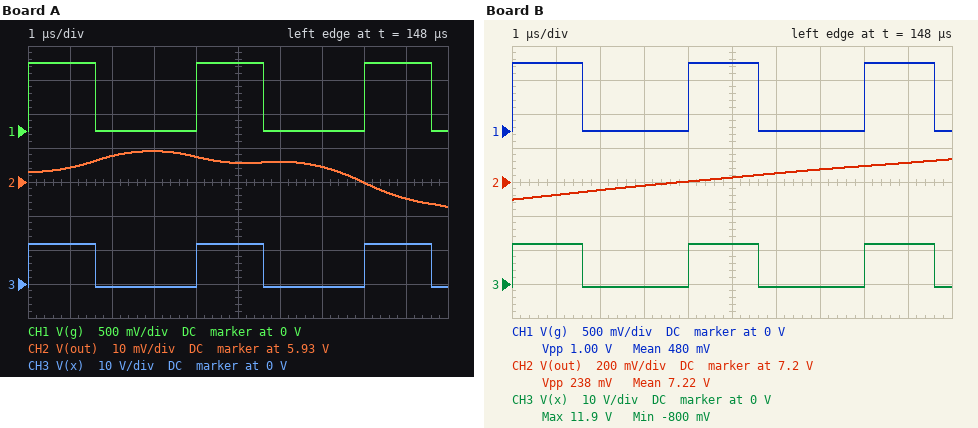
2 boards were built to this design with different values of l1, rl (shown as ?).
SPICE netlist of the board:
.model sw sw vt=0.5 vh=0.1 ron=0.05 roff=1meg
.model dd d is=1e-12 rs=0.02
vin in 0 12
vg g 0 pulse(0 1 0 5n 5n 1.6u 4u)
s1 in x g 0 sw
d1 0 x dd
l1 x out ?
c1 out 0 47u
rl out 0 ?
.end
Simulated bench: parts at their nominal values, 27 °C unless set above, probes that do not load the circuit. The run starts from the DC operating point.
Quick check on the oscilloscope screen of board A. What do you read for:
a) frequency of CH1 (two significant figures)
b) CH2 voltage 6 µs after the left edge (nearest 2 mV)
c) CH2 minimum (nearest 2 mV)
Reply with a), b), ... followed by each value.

a) 250 kHz
b) 5.936 V
c) 5.922 V
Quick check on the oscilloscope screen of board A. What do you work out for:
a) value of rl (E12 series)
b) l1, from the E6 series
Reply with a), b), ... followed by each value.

a) 1.8 Ω
b) 47 µH
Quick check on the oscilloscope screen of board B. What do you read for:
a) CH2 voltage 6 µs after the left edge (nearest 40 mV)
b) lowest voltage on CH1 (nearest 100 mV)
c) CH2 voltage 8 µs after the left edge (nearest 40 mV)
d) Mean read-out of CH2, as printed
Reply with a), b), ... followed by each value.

a) 7.24 V
b) 0 V
c) 7.28 V
d) 7.22 V
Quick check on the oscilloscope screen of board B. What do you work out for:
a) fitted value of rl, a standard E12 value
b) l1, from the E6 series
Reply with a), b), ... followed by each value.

a) 6.8 Ω
b) 68 µH
